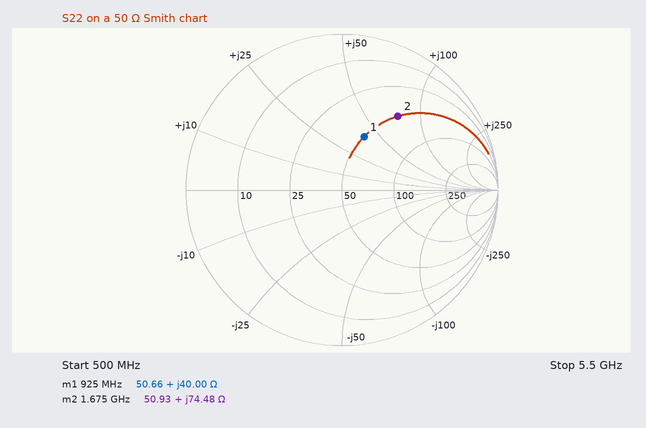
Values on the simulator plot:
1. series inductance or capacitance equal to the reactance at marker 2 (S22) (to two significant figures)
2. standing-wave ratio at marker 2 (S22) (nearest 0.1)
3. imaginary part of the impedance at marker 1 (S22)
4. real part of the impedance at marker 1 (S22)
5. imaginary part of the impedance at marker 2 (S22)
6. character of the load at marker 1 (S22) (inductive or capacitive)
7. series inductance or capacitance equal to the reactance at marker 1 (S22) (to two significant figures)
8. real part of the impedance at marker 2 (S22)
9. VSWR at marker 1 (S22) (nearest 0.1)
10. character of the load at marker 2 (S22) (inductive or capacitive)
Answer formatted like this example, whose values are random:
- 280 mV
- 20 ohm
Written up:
- 7.1 nH
- 3.9
- +40.00 Ω
- 50.66 Ω
- +74.48 Ω
- inductive
- 6.9 nH
- 50.93 Ω
- 2.2
- inductive
